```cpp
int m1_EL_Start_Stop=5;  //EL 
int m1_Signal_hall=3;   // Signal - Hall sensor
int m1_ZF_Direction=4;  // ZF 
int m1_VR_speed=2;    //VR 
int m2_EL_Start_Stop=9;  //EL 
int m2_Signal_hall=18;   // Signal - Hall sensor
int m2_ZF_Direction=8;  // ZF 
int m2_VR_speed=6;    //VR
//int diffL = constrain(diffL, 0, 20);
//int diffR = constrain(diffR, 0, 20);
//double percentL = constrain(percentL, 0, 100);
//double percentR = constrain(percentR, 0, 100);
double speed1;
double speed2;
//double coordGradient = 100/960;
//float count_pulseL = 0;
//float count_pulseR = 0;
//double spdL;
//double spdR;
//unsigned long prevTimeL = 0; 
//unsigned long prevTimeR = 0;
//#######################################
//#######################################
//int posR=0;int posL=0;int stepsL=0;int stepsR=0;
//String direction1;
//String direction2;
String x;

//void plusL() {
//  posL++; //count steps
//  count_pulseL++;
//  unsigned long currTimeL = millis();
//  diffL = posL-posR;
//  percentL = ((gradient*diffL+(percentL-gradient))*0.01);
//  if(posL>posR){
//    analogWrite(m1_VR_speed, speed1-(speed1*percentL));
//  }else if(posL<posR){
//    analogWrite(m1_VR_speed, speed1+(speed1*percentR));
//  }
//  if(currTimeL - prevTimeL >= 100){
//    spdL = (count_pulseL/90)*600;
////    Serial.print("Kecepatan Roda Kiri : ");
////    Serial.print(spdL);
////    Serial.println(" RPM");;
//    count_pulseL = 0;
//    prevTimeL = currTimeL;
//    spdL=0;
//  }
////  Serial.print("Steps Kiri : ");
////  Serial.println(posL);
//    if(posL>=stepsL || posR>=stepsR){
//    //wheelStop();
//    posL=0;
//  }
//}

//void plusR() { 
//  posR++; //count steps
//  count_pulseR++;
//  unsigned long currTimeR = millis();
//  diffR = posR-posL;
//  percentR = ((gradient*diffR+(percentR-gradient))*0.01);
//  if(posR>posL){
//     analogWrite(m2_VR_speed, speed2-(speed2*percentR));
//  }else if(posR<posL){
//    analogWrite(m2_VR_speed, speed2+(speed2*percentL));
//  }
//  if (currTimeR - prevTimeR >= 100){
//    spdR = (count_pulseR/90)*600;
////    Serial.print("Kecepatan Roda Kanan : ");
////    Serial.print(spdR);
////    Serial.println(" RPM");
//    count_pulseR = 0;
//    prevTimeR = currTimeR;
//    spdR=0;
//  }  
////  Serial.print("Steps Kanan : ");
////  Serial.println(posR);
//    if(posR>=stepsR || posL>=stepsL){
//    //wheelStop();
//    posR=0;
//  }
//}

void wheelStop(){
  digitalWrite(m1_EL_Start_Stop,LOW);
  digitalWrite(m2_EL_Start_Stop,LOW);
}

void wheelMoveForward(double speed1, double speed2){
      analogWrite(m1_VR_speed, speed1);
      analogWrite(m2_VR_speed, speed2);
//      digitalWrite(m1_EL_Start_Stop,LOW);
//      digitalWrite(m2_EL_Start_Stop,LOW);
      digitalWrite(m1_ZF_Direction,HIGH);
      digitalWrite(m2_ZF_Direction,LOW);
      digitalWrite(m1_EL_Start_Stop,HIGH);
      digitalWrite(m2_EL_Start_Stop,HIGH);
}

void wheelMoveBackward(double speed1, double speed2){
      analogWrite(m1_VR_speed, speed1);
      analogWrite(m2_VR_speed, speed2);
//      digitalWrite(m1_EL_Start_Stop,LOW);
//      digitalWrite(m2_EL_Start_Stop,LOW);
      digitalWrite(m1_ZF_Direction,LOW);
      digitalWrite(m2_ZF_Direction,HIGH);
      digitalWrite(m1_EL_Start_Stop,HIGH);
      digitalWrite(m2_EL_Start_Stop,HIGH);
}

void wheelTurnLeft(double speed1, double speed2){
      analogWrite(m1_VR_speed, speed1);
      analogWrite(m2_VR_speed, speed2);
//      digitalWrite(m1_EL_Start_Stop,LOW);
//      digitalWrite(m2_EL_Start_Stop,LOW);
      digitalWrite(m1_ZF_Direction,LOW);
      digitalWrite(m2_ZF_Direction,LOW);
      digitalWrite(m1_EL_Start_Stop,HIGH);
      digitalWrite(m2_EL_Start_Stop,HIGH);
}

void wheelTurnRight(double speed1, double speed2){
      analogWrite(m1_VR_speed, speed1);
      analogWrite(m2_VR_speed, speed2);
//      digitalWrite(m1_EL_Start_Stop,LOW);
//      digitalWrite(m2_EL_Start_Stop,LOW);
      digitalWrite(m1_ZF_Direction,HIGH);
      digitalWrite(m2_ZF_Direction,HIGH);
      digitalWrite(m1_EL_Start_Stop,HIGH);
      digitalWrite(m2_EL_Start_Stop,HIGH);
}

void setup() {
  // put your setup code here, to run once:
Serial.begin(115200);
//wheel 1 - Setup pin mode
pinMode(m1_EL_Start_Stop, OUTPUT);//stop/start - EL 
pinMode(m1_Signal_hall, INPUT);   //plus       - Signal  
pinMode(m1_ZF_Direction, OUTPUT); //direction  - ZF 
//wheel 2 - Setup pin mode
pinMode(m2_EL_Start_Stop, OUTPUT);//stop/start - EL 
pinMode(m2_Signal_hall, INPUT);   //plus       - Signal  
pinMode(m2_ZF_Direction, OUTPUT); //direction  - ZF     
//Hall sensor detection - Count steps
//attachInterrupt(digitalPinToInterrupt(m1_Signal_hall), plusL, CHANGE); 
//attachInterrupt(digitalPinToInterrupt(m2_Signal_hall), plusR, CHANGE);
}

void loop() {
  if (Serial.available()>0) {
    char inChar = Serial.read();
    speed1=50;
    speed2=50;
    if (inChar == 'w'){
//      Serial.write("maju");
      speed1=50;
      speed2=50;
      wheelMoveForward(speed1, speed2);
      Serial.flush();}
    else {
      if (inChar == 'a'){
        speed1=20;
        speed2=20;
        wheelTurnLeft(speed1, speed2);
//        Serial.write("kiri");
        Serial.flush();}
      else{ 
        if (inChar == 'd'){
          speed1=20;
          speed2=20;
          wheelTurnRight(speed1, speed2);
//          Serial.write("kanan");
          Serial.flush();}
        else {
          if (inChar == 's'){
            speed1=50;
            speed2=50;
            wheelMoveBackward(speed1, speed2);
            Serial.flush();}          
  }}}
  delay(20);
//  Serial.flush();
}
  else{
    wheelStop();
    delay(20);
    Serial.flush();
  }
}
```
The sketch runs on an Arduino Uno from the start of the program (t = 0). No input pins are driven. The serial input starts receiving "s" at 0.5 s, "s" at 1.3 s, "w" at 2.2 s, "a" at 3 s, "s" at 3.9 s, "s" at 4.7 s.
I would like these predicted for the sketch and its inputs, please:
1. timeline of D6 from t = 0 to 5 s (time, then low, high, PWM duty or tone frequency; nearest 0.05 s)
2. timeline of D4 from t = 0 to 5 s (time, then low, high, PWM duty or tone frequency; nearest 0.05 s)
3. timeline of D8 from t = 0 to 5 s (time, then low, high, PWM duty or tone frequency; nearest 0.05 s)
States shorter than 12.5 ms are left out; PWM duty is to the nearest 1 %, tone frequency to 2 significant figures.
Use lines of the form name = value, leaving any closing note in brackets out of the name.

timeline of D6 from t = 0 to 5 s = 0.5 s PWM 20 %; 3 s PWM 8 %; 3.9 s PWM 20 %
timeline of D4 from t = 0 to 5 s = 0 s low; 2.2 s high; 3 s low
timeline of D8 from t = 0 to 5 s = 0 s low; 0.5 s high; 2.2 s low; 3.9 s high
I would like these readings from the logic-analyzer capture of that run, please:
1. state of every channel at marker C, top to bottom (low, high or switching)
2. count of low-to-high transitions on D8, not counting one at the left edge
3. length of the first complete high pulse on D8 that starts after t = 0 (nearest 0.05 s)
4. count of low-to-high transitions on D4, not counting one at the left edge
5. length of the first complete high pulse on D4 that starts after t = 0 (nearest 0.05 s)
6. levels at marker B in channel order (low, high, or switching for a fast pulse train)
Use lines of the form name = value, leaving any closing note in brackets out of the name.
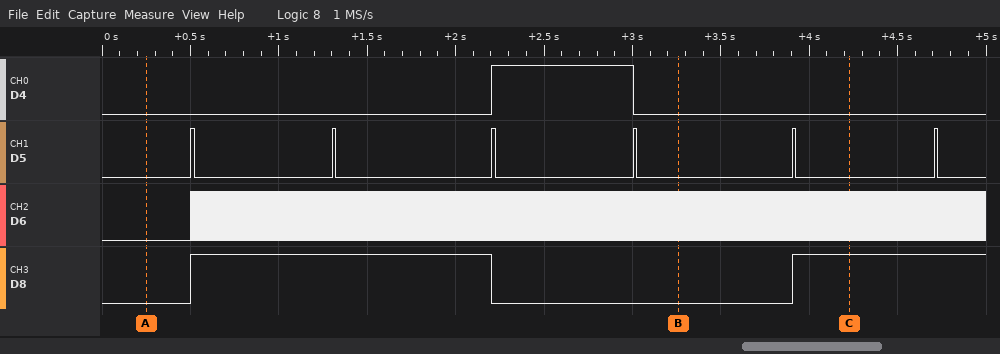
state of every channel at marker C, top to bottom = D4 low, D5 low, D6 switching, D8 high
count of low-to-high transitions on D8, not counting one at the left edge = 2
length of the first complete high pulse on D8 that starts after t = 0 = 1.70 s
count of low-to-high transitions on D4, not counting one at the left edge = 1
length of the first complete high pulse on D4 that starts after t = 0 = 0.80 s
levels at marker B in channel order = D4 low, D5 low, D6 switching, D8 low
